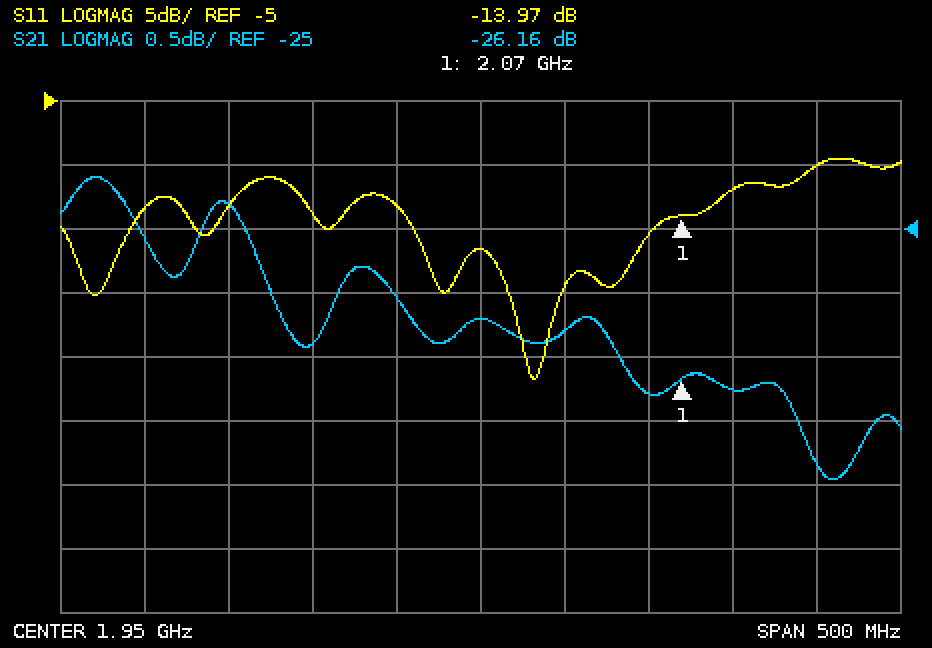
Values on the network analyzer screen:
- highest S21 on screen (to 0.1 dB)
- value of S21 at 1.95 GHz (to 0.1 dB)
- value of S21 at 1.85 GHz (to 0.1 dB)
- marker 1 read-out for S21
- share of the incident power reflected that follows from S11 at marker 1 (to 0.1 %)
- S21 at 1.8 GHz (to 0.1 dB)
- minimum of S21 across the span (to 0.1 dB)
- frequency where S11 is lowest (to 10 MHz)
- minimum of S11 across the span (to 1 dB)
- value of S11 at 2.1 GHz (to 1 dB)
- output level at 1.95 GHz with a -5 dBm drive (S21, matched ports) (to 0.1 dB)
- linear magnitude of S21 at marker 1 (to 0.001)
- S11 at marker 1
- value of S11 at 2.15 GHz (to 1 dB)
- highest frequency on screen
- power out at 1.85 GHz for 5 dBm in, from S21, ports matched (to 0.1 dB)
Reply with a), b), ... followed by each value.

a) -24.6 dB
b) -25.7 dB
c) -25.9 dB
d) -26.16 dB
e) 4.0 %
f) -24.8 dB
g) -27.0 dB
h) 1.98 GHz
i) -27 dB
j) -12 dB
k) -30.7 dBm
l) 0.049
m) -13.97 dB
n) -10 dB
o) 2.2 GHz
p) -20.9 dBm
